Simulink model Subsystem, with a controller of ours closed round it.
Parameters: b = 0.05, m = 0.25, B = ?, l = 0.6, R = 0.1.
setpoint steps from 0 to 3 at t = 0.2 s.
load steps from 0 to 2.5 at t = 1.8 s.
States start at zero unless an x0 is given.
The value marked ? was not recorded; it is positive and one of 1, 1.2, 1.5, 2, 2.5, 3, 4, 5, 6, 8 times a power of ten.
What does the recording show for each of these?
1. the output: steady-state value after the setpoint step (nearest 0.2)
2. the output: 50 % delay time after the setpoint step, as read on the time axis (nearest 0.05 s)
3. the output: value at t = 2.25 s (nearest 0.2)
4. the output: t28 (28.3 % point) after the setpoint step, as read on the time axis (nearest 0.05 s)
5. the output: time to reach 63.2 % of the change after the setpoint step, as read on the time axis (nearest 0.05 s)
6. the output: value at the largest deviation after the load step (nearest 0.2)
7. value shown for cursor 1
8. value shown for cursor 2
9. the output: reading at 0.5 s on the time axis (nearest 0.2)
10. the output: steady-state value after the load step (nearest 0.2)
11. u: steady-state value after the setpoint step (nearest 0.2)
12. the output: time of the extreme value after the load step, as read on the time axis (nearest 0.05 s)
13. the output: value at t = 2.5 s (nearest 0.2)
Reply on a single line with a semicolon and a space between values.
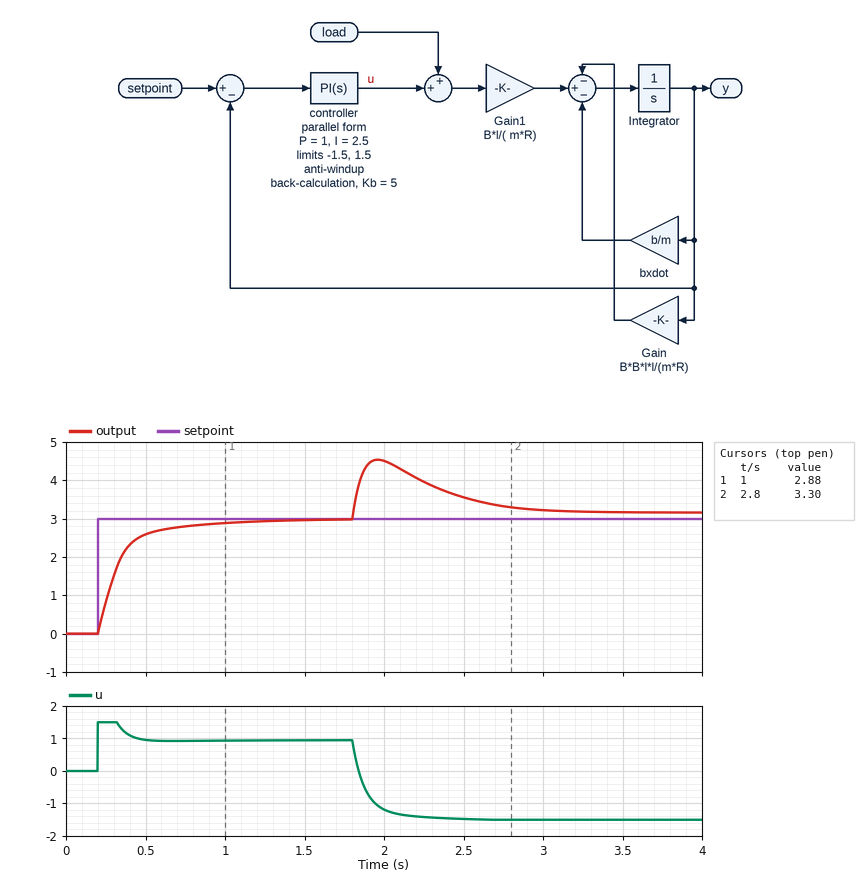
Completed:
3.0; 0.30 s; 4.0; 0.25 s; 0.35 s; 4.6; 2.88; 3.30; 2.6; 3.2; 1.0; 1.95 s; 3.6
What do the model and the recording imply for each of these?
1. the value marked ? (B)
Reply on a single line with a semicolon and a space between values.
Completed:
0.5
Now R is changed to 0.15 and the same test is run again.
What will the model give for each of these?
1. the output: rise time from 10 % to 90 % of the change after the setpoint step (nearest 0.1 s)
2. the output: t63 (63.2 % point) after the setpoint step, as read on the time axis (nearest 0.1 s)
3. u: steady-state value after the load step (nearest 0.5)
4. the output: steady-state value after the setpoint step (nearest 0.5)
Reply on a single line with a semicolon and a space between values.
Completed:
0.4 s; 0.4 s; -1.5; 3.0
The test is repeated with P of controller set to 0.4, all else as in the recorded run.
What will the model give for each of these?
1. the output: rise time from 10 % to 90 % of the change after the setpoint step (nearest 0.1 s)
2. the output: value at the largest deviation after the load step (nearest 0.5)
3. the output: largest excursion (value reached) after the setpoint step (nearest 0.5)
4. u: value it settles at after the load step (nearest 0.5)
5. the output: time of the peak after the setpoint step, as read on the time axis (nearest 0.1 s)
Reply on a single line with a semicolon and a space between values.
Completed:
0.3 s; 5.5; 3.0; -1.5; 0.8 s
